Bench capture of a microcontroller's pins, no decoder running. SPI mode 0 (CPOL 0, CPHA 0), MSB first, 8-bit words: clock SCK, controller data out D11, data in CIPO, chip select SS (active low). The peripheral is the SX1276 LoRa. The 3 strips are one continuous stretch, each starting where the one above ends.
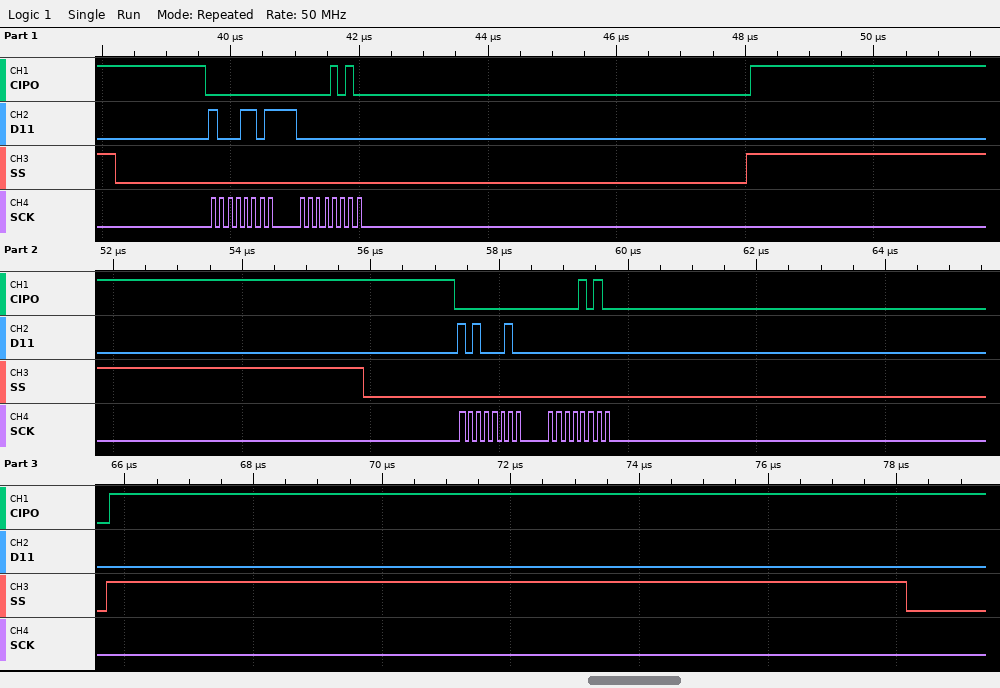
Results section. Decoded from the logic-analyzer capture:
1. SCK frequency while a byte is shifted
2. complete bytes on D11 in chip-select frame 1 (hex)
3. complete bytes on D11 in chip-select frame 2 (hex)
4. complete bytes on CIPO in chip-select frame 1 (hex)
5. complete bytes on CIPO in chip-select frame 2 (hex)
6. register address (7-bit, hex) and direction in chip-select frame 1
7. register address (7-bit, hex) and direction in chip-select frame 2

8 MHz
8D 00
A2 00
00 0A
00 0A
0x0D write
0x22 write
